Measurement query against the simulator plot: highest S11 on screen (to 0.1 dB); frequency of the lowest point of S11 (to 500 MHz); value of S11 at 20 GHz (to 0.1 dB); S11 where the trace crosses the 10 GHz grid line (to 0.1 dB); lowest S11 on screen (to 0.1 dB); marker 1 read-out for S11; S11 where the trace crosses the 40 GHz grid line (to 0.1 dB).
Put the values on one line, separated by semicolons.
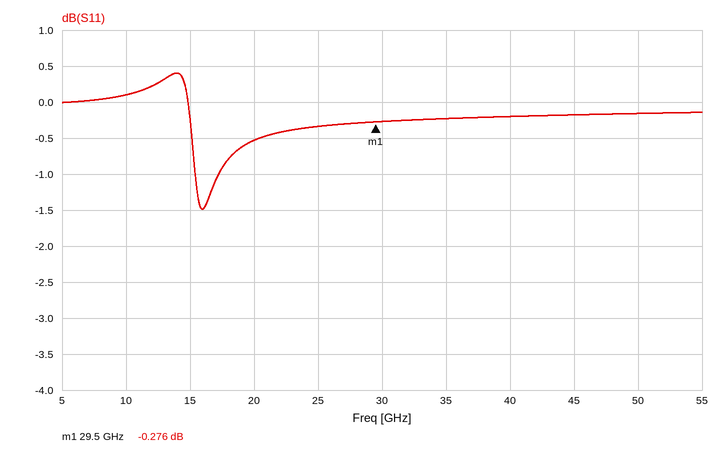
0.4 dB; 16.0 GHz; -0.5 dB; 0.1 dB; -1.5 dB; -0.276 dB; -0.2 dB
